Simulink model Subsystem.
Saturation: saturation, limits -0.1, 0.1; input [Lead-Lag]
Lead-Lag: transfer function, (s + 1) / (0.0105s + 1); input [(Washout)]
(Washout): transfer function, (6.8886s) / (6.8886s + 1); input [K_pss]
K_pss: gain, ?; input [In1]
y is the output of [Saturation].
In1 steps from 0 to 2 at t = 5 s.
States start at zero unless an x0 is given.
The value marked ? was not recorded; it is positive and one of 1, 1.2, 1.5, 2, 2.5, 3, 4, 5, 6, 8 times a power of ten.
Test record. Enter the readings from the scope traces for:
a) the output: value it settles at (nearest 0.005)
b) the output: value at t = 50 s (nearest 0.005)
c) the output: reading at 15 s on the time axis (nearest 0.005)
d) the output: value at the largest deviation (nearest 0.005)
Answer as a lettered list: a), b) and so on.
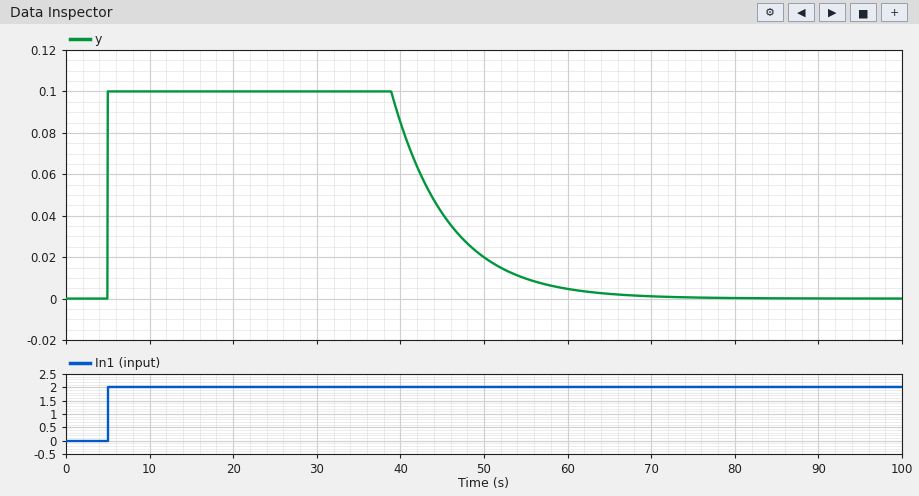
a) 0.000
b) 0.020
c) 0.100
d) 0.100
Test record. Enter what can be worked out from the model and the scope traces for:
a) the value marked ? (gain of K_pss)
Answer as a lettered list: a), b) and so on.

a) 8
